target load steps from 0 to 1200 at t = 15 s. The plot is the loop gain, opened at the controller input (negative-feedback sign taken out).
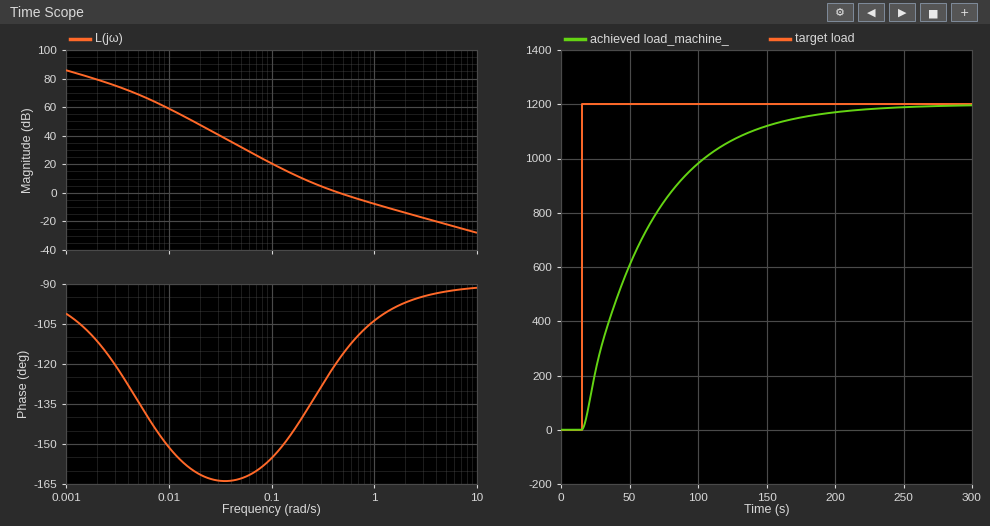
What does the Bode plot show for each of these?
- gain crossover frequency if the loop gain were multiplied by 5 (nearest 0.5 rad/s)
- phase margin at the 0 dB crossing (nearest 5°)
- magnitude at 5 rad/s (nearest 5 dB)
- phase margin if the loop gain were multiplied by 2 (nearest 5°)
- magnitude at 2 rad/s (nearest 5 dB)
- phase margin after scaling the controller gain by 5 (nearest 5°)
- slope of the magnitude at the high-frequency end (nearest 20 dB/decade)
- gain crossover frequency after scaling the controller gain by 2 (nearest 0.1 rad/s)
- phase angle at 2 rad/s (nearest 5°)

2.0 rad/s
60°
-20 dB
75°
-15 dB
85°
-20 dB/decade
0.8 rad/s
-95°
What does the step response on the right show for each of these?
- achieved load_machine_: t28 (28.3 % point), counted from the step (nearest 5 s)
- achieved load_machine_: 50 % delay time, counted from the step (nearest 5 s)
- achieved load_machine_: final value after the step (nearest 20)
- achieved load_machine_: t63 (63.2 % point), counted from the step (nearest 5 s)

15 s
35 s
1200
50 s
